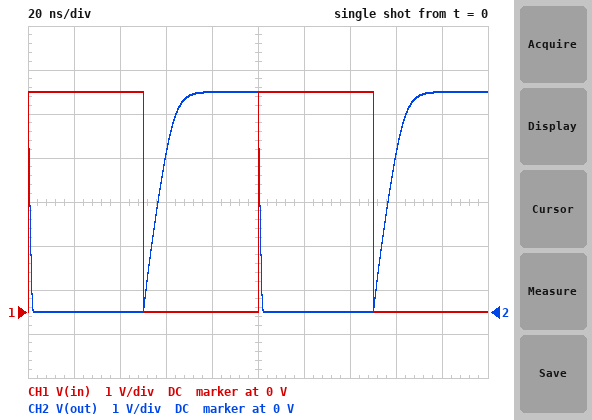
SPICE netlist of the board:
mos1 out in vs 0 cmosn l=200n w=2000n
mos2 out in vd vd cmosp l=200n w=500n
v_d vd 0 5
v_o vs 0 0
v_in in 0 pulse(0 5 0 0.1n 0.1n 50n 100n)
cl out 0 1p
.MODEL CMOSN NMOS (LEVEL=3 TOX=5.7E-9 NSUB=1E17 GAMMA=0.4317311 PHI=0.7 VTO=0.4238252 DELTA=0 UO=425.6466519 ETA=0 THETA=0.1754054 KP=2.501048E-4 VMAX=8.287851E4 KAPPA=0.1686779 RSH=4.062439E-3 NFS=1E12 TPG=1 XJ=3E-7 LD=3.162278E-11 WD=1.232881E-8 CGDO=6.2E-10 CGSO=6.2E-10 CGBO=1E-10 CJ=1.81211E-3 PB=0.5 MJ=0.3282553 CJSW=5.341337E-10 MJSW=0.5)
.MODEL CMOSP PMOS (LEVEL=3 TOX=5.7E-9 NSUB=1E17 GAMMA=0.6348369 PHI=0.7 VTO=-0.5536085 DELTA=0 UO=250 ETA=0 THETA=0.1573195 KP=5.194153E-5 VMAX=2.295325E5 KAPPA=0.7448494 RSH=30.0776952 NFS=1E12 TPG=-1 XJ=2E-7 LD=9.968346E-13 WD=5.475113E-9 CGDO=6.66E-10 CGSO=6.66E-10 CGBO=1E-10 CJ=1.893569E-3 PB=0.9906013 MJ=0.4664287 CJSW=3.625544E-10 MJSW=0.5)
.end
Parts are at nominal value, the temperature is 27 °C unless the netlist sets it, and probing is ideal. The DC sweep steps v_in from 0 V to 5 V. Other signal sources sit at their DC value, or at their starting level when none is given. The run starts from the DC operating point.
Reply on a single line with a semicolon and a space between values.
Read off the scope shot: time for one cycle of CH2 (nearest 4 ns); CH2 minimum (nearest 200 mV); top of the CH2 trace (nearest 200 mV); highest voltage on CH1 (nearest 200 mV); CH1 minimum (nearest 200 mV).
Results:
100 ns; 0 V; 5.0 V; 5.0 V; 0 V
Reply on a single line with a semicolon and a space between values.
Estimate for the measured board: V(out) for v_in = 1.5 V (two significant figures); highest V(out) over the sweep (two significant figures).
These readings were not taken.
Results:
180 mV; 5.0 V
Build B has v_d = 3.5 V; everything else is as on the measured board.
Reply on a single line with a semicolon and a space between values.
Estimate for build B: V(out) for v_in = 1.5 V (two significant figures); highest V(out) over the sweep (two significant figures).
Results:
49 mV; 3.5 V
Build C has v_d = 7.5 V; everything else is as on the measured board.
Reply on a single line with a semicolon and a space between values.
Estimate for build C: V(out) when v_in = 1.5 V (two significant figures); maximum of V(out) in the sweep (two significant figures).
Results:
1.9 V; 7.5 V
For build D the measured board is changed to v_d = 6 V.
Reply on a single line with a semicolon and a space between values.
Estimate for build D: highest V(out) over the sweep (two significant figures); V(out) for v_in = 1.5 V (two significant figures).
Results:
6.0 V; 420 mV
